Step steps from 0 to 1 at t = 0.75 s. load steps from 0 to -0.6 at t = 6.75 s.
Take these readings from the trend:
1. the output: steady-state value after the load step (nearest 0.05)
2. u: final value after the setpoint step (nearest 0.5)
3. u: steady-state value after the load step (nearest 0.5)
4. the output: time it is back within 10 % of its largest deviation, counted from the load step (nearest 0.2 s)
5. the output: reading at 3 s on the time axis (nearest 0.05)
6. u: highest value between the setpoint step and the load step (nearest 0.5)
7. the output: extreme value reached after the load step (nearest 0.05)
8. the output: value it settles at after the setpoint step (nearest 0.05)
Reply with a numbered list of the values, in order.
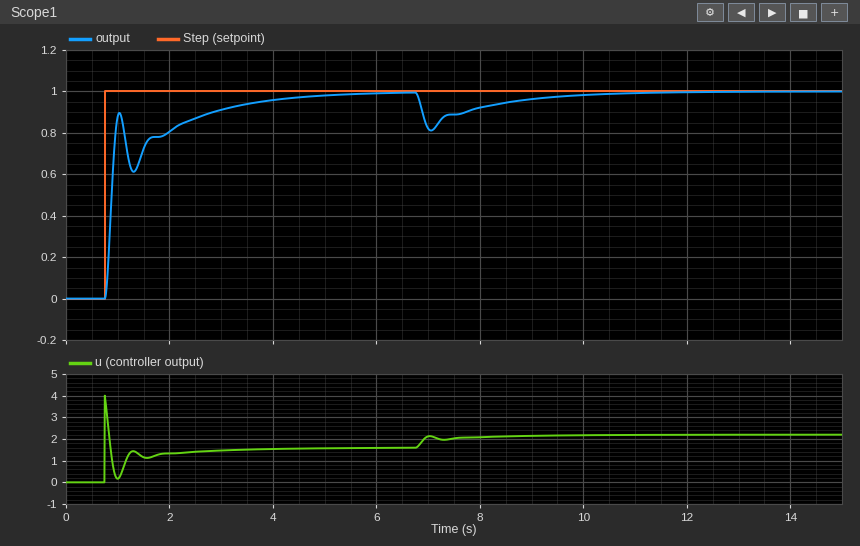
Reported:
1. 1.00
2. 1.5
3. 2.0
4. 3.2 s
5. 0.90
6. 4.0
7. 0.80
8. 1.00
